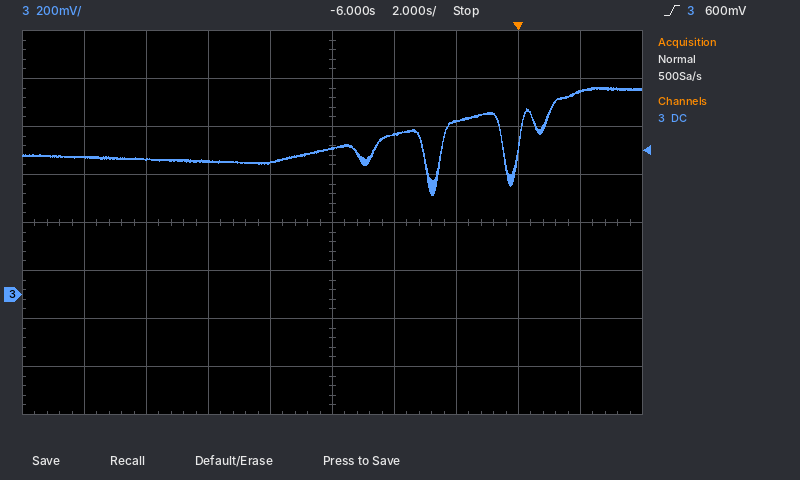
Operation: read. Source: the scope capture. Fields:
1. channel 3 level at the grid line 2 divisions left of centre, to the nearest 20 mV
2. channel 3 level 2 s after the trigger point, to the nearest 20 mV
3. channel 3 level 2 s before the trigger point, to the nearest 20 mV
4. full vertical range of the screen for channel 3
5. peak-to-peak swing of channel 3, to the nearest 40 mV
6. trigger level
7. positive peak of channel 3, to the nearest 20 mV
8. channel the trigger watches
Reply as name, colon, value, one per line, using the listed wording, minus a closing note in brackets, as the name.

channel 3 level at the grid line 2 divisions left of centre, to the nearest 20 mV: 560 mV
channel 3 level 2 s after the trigger point, to the nearest 20 mV: 840 mV
channel 3 level 2 s before the trigger point, to the nearest 20 mV: 720 mV
full vertical range of the screen for channel 3: 1.6 V
peak-to-peak swing of channel 3, to the nearest 40 mV: 440 mV
trigger level: 600 mV
positive peak of channel 3, to the nearest 20 mV: 860 mV
channel the trigger watches: channel 3
